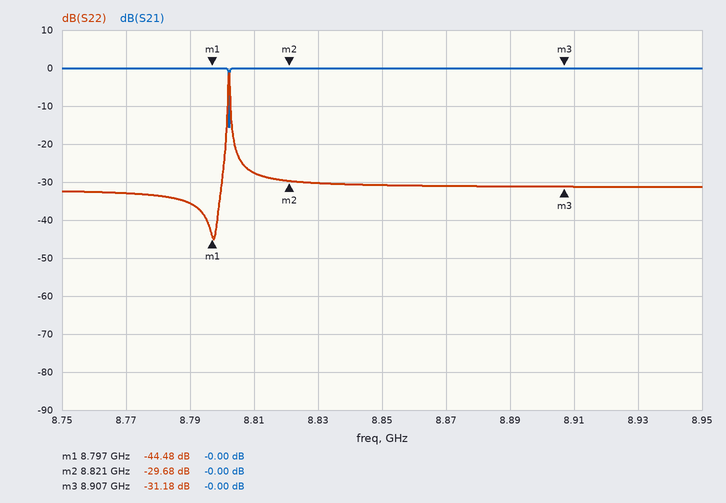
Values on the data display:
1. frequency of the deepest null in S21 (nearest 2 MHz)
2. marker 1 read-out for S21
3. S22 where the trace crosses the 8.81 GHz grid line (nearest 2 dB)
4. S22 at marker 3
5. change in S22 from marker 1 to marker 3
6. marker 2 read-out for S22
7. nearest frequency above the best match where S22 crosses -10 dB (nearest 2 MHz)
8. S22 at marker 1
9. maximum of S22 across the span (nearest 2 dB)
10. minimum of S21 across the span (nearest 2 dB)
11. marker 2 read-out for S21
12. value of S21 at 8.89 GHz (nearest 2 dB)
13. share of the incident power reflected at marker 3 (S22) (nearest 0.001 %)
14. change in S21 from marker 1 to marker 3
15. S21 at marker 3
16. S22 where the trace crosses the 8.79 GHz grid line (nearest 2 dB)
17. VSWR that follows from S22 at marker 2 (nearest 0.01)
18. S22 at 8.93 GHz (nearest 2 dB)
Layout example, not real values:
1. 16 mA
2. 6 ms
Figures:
1. 8.802 GHz
2. -0.00 dB
3. -28 dB
4. -31.18 dB
5. 13.30 dB
6. -29.68 dB
7. 8.802 GHz
8. -44.48 dB
9. -2 dB
10. -16 dB
11. -0.00 dB
12. 0 dB
13. 0.076 %
14. 0.00 dB
15. -0.00 dB
16. -36 dB
17. 1.07
18. -32 dB
